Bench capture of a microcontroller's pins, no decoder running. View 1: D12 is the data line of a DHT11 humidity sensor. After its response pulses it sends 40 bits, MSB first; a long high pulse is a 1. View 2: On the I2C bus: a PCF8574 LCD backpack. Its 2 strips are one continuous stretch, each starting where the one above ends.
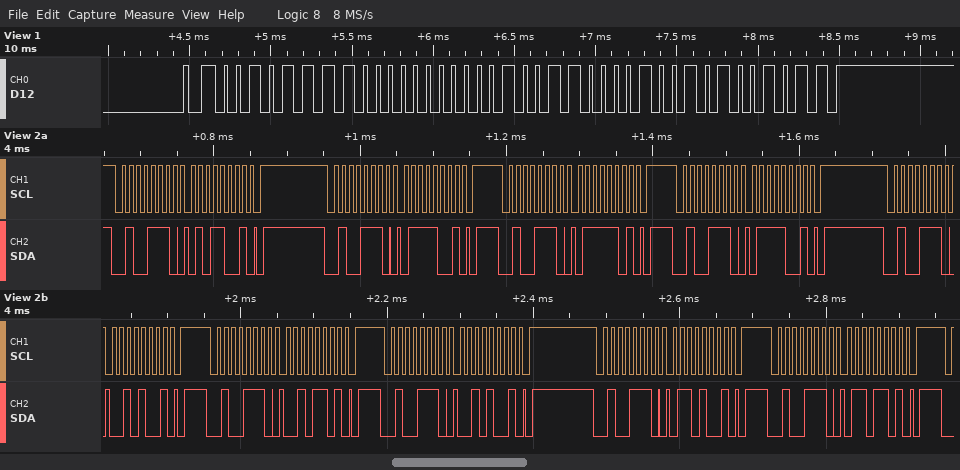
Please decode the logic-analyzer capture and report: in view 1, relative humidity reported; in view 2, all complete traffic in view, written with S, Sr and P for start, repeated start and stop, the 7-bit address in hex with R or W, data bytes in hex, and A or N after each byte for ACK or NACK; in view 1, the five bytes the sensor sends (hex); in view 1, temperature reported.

47 %
S 27W A 59 A P S 27W A 79 A P S 27W A 7D A P S 27W A 79 A P S 27W A 29 A P S 27W A 2D A P S 27W A 29 A P S 27W A 69 A P S 27W A 6D A P
2F 00 13 09 4B
19.9 °C
